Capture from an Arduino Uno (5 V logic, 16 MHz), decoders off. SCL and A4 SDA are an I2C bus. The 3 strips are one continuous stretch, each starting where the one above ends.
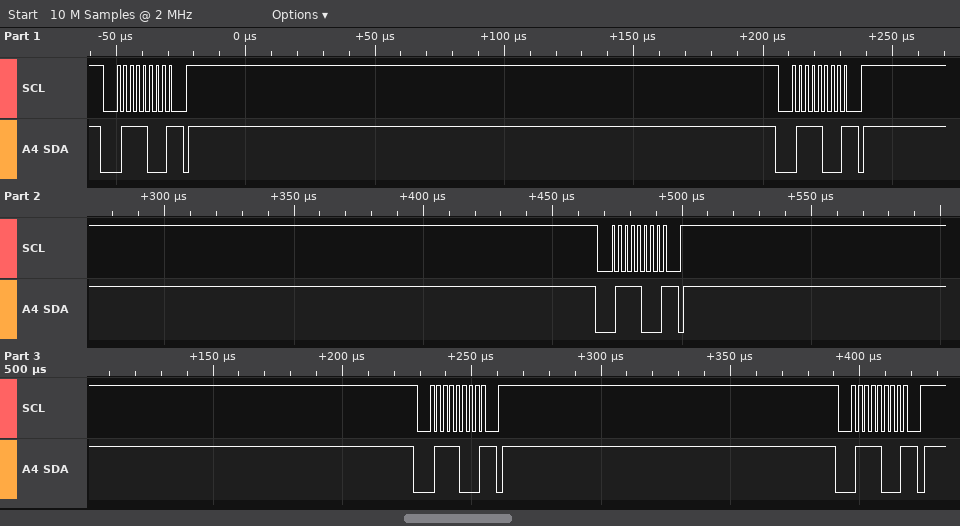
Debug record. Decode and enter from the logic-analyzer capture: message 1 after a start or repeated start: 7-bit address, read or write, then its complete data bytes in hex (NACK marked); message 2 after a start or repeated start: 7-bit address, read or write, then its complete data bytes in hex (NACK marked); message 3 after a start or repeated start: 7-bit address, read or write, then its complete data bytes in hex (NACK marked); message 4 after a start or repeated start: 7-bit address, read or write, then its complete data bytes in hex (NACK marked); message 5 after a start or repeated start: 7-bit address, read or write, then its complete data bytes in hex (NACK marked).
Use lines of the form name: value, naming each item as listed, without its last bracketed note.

message 1 after a start or repeated start: 7-bit address, read or write, then its complete data bytes in hex: 0x3C write NACK
message 2 after a start or repeated start: 7-bit address, read or write, then its complete data bytes in hex: 0x3C write NACK
message 3 after a start or repeated start: 7-bit address, read or write, then its complete data bytes in hex: 0x3C write NACK
message 4 after a start or repeated start: 7-bit address, read or write, then its complete data bytes in hex: 0x3C write NACK
message 5 after a start or repeated start: 7-bit address, read or write, then its complete data bytes in hex: 0x3C write NACK
